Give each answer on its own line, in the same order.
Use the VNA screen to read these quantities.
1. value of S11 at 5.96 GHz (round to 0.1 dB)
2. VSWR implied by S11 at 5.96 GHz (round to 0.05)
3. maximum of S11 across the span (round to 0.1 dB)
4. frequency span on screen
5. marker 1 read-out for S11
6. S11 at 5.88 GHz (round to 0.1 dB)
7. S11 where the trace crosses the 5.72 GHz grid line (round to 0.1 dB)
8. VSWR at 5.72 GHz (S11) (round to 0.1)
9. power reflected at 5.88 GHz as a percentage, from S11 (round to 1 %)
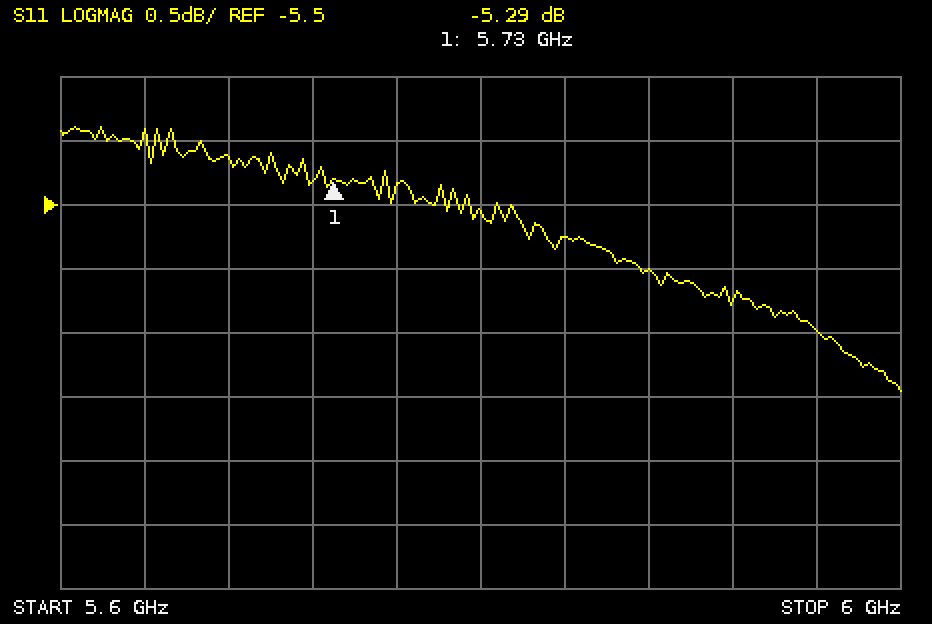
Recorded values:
-6.5 dB
2.80
-4.9 dB
400 MHz
-5.29 dB
-6.0 dB
-5.3 dB
3.4
25 %
